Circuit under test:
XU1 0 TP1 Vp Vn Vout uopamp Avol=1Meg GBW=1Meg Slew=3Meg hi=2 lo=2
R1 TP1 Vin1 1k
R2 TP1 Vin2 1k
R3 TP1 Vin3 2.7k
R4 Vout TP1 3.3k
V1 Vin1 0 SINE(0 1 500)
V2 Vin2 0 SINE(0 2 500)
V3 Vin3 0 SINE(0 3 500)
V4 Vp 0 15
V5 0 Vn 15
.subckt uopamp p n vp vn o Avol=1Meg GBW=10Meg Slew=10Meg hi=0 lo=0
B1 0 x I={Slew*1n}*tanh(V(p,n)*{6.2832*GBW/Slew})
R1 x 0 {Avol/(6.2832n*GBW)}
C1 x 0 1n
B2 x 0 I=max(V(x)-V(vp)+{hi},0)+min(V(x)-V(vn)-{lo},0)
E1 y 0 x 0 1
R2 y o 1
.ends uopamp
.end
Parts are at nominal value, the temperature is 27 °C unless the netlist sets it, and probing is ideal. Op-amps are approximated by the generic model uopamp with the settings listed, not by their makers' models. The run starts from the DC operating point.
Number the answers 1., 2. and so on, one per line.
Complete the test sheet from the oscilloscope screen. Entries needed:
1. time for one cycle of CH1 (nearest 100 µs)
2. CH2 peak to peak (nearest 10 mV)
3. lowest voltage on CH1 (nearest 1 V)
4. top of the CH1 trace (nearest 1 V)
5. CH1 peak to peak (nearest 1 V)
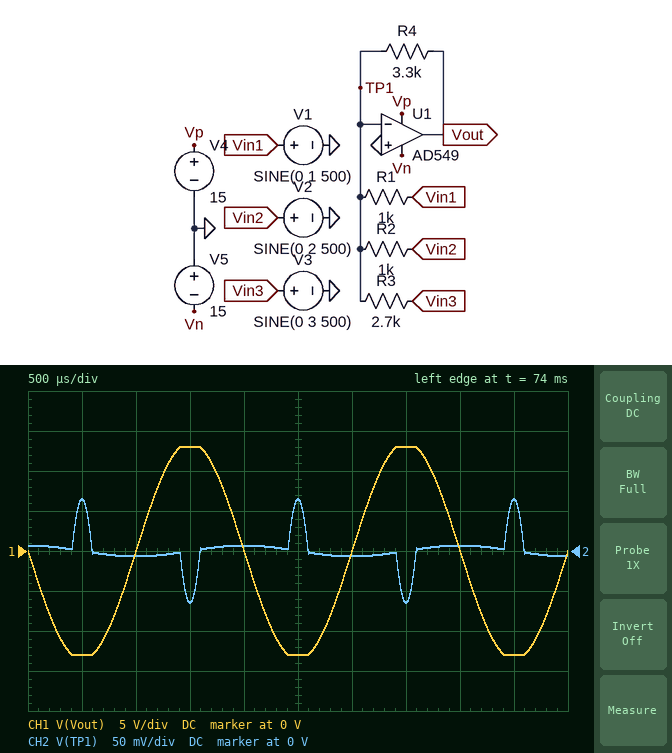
1. 2.0 ms
2. 130 mV
3. -13 V
4. 13 V
5. 26 V
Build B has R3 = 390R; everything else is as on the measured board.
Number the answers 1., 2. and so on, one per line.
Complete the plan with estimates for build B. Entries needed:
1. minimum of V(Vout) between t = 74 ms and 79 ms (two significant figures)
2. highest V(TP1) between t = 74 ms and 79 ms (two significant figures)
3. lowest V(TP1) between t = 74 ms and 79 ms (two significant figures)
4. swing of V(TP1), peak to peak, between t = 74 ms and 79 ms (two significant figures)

1. -13 V
2. 1.4 V
3. -1.4 V
4. 2.8 V
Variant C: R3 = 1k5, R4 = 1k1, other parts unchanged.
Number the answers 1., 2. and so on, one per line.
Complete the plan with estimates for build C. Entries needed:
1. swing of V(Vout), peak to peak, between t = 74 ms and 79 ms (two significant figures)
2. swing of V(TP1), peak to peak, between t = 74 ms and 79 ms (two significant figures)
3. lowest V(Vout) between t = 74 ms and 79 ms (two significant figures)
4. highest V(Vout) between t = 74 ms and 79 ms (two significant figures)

1. 11 V
2. 5.5 mV
3. -5.5 V
4. 5.5 V
